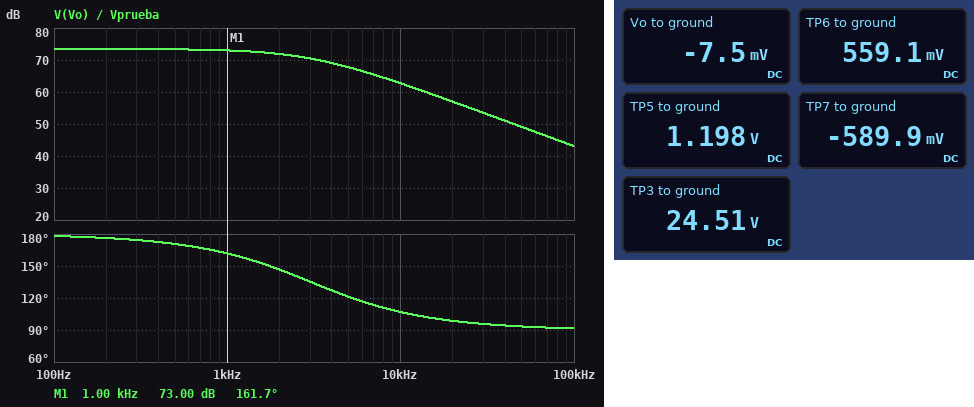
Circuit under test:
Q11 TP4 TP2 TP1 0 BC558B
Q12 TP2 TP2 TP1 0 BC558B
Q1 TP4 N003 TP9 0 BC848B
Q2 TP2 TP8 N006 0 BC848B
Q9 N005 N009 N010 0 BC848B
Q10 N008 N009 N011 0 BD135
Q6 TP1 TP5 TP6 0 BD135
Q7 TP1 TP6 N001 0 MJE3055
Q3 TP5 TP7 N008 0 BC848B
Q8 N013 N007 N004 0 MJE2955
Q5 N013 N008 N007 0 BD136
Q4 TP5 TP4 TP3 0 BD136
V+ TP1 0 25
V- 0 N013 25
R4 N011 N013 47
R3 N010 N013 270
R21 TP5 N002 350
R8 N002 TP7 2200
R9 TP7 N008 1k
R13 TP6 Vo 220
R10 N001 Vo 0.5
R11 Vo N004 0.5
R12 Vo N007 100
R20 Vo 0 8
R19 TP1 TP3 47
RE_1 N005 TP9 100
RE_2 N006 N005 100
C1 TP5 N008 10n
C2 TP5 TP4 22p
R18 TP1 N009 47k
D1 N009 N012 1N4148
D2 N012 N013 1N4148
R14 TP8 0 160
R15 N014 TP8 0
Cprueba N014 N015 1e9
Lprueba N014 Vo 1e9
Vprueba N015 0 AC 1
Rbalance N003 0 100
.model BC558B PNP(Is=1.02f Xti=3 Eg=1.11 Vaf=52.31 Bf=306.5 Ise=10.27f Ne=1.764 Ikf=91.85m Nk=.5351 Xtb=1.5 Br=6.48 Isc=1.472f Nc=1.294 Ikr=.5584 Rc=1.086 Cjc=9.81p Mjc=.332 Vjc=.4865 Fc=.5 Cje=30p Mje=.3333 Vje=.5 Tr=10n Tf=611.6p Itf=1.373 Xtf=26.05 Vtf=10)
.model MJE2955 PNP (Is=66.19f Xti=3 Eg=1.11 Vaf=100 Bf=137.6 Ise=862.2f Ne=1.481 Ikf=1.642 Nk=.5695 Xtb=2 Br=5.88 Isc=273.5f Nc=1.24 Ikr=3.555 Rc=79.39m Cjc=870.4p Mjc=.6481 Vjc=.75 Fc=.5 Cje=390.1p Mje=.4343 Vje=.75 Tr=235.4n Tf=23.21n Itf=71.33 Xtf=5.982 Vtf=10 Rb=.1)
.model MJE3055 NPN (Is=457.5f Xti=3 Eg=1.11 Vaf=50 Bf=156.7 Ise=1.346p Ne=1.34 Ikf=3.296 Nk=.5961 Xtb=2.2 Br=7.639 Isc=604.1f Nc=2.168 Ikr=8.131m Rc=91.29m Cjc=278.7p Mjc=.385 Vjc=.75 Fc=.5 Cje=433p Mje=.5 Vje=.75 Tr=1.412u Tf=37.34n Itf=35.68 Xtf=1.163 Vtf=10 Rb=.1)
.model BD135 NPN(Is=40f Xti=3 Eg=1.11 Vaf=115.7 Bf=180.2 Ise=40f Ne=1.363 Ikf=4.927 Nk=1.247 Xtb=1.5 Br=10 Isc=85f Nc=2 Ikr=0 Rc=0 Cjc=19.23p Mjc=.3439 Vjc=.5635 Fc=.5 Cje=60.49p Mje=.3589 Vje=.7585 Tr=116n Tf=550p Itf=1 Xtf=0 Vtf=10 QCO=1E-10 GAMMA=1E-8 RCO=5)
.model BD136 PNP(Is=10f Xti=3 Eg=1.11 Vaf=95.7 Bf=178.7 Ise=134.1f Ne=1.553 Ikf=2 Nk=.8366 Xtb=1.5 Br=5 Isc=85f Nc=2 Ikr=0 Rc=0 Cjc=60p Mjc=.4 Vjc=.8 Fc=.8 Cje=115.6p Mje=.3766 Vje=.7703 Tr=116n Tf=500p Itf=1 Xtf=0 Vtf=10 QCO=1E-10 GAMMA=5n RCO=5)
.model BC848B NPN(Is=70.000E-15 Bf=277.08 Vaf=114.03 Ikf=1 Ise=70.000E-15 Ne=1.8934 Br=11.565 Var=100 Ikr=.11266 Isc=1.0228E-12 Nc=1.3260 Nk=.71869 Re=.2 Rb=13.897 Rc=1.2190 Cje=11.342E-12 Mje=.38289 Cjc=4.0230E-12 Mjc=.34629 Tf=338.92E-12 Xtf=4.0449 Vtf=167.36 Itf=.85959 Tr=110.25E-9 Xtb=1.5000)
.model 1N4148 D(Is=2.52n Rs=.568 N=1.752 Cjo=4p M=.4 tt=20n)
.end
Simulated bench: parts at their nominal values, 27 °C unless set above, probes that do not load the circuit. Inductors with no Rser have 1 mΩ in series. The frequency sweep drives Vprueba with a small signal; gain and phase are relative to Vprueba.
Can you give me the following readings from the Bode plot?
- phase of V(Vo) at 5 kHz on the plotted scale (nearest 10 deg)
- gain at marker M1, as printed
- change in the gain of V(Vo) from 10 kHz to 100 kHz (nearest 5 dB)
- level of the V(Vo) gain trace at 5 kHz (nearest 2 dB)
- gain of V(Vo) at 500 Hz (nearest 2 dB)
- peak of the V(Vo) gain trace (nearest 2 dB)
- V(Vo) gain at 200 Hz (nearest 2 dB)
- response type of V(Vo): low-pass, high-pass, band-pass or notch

120 deg
73.00 dB
-20 dB
68 dB
74 dB
74 dB
74 dB
low-pass
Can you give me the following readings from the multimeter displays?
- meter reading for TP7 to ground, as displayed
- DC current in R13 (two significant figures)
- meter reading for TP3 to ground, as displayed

-589.9 mV
2.6 mA
24.51 V
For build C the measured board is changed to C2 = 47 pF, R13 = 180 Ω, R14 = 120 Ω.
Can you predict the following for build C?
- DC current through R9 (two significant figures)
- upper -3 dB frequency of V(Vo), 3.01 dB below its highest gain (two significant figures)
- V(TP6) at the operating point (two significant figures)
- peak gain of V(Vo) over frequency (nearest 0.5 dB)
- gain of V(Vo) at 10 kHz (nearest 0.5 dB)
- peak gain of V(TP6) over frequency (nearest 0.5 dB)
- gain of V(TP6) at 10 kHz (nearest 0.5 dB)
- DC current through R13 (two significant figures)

670 µA
1.9 kHz
550 mV
72.0 dB
57.5 dB
80.0 dB
65.5 dB
3.1 mA
